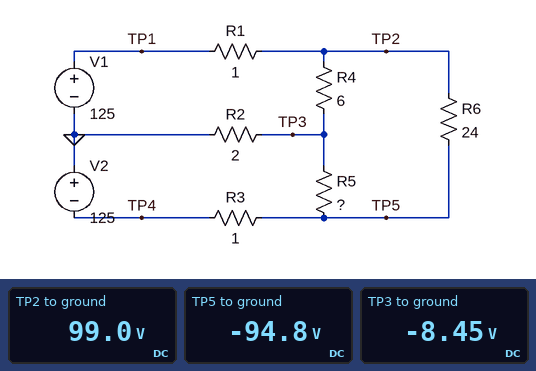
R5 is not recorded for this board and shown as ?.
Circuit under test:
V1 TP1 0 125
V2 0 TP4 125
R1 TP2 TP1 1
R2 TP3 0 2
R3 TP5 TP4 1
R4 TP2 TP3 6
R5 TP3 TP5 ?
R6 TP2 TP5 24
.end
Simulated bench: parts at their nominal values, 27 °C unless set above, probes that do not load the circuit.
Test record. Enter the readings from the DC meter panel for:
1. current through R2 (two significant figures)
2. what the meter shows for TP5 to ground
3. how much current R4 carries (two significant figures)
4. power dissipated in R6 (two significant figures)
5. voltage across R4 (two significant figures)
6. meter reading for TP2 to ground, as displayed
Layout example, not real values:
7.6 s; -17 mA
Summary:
4.2 A; -94.8 V; 18 A; 1.6 kW; 110 V; 99.0 V
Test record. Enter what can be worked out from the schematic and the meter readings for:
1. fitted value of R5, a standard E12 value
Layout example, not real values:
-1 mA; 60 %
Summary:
3.9 Ω
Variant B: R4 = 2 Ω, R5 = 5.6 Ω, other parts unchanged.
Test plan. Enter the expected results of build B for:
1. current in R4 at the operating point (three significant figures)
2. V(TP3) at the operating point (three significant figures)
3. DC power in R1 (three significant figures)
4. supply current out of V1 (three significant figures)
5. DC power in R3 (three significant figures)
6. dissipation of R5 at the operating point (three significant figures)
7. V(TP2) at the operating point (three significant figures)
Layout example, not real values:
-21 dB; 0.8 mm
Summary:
31.9 A; 21.7 V; 1.56 kW; 39.5 A; 821 W; 2.49 kW; 85.5 V
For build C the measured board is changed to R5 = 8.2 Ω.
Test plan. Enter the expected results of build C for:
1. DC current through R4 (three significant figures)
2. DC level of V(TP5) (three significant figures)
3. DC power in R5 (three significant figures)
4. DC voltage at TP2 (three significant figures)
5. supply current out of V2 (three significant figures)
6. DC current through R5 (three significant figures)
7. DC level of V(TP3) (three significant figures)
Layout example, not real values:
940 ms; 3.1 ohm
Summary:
15.9 A; -103 V; 1.44 kW; 101 V; 21.7 A; 13.2 A; 5.30 V
